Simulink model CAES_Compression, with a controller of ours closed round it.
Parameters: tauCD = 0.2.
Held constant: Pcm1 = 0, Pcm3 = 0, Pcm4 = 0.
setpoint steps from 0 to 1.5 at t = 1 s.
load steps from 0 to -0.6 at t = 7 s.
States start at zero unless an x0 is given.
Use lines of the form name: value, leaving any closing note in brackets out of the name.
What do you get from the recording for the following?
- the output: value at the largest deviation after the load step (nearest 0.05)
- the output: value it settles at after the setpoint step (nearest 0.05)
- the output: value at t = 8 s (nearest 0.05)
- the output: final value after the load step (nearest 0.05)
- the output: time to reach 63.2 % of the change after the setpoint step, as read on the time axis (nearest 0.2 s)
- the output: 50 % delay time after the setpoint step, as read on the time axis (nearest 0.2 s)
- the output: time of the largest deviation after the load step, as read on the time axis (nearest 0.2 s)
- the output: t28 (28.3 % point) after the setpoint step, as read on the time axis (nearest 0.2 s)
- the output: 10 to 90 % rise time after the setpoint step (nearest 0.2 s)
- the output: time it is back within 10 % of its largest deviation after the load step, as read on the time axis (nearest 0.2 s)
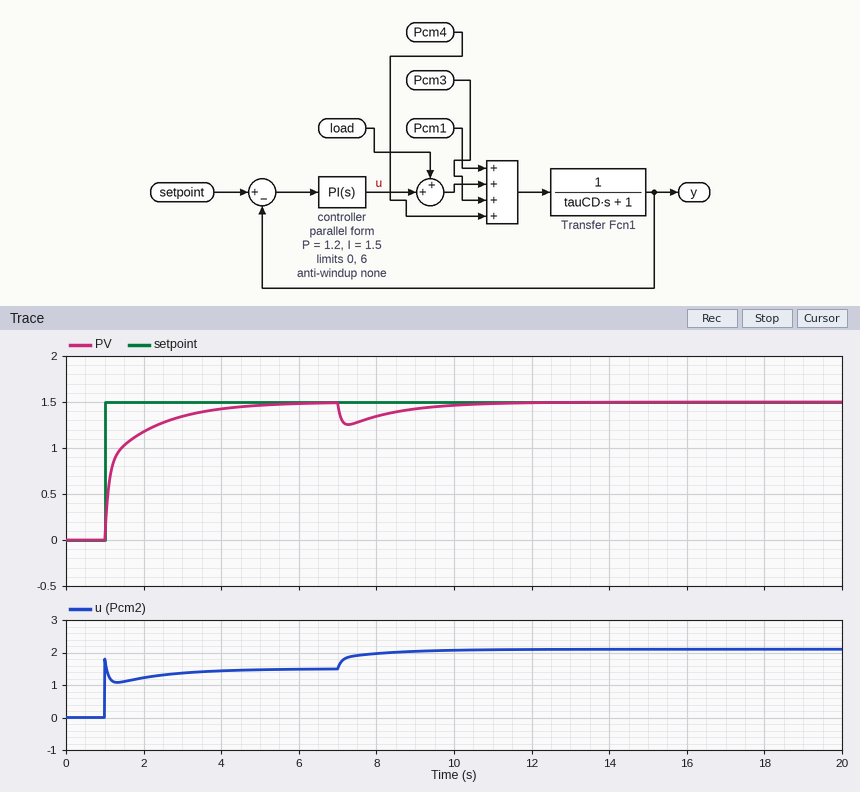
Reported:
the output: value at the largest deviation after the load step: 1.25
the output: value it settles at after the setpoint step: 1.50
the output: value at t = 8 s: 1.35
the output: final value after the load step: 1.50
the output: time to reach 63.2 % of the change after the setpoint step, as read on the time axis: 1.4 s
the output: 50 % delay time after the setpoint step, as read on the time axis: 1.2 s
the output: time of the largest deviation after the load step, as read on the time axis: 7.2 s
the output: t28 (28.3 % point) after the setpoint step, as read on the time axis: 1.0 s
the output: 10 to 90 % rise time after the setpoint step: 2.0 s
the output: time it is back within 10 % of its largest deviation after the load step, as read on the time axis: 10.6 s
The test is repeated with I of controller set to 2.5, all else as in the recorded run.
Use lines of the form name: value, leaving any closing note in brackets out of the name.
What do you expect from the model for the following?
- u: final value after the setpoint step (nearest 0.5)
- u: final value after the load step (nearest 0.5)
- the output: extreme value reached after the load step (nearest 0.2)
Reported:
u: final value after the setpoint step: 1.5
u: final value after the load step: 2.0
the output: extreme value reached after the load step: 1.2
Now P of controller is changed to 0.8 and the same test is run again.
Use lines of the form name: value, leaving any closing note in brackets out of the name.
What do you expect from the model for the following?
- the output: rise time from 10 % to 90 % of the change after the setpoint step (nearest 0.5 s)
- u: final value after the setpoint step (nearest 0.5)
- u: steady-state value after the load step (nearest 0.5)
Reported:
the output: rise time from 10 % to 90 % of the change after the setpoint step: 2.0 s
u: final value after the setpoint step: 1.5
u: steady-state value after the load step: 2.0
